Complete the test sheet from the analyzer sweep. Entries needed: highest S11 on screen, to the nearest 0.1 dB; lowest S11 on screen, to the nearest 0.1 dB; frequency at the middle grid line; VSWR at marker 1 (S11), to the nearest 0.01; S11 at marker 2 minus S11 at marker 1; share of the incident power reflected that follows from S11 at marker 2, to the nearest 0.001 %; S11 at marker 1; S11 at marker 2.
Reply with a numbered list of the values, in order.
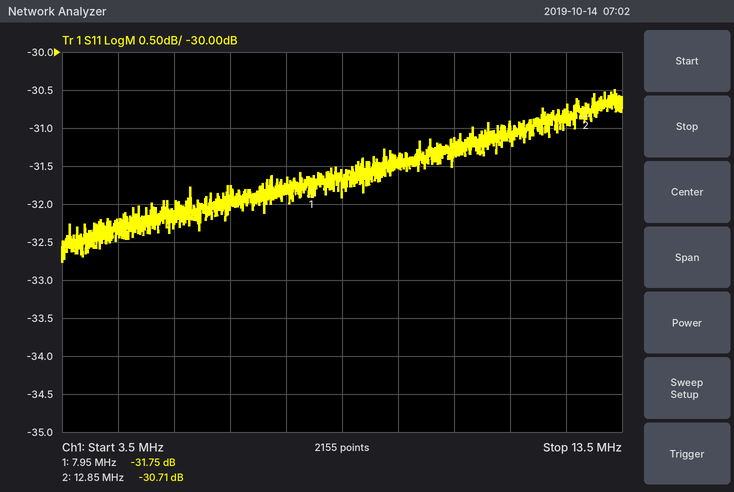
1. -30.5 dB
2. -32.8 dB
3. 8.5 MHz
4. 1.05
5. 1.04 dB
6. 0.085 %
7. -31.75 dB
8. -30.71 dB
